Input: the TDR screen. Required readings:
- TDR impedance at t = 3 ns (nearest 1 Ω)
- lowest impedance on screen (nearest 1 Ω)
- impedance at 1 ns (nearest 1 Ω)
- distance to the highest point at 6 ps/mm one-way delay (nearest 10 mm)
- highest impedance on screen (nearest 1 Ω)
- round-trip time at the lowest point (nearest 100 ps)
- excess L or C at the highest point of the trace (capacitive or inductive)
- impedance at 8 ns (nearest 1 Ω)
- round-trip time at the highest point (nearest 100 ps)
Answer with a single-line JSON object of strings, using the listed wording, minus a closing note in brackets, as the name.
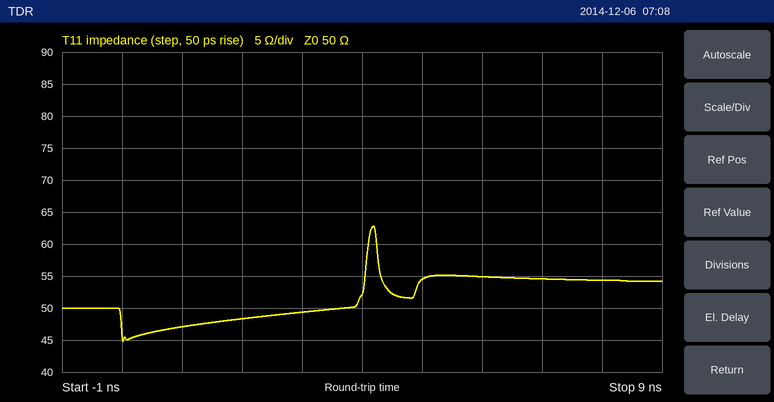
{"TDR impedance at t = 3 ns": "49 Ω", "lowest impedance on screen": "45 Ω", "impedance at 1 ns": "47 Ω", "distance to the highest point at 6 ps/mm one-way delay": "350 mm", "highest impedance on screen": "63 Ω", "round-trip time at the lowest point": "0.0 ns", "excess L or C at the highest point of the trace": "inductive", "impedance at 8 ns": "54 Ω", "round-trip time at the highest point": "4.2 ns"}
